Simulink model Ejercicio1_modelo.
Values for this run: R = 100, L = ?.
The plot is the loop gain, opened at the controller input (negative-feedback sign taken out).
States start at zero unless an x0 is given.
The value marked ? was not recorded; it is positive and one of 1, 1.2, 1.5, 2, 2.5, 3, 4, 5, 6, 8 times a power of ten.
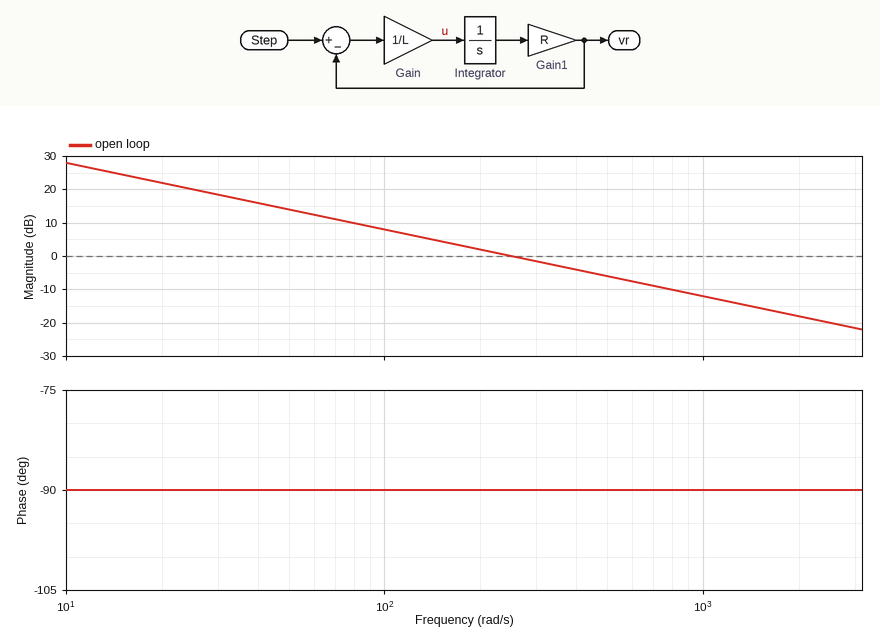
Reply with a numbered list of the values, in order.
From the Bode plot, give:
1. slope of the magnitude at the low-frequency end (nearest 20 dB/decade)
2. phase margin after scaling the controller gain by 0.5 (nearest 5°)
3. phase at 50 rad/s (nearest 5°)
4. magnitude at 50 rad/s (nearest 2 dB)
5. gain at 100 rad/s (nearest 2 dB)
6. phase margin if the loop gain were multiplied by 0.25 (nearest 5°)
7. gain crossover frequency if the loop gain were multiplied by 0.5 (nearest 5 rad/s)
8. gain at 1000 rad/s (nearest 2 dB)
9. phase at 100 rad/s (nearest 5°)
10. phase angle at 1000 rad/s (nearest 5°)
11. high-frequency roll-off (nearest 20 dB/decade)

1. -20 dB/decade
2. 90°
3. -90°
4. 14 dB
5. 8 dB
6. 90°
7. 125 rad/s
8. -12 dB
9. -90°
10. -90°
11. -20 dB/decade
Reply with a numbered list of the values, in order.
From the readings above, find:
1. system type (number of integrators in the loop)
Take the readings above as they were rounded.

1. 1
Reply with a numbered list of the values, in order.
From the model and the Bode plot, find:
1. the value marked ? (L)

1. 0.4
